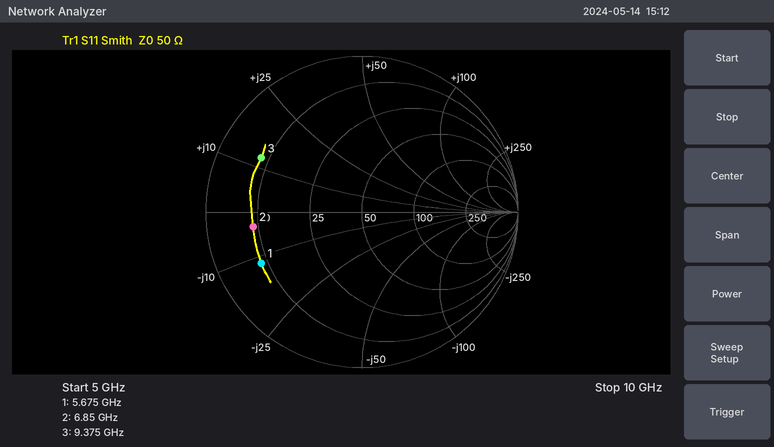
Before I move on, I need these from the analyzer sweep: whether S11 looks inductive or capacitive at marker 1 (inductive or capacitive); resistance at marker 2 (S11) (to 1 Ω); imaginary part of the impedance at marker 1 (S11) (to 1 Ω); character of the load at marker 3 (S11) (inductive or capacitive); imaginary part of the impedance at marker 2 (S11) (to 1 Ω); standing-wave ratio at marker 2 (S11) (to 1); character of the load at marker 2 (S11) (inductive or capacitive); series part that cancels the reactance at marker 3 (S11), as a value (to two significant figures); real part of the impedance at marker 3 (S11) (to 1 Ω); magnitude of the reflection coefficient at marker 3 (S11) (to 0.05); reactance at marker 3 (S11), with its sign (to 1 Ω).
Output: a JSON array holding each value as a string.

["capacitive", "9 Ω", "-12 Ω", "inductive", "-3 Ω", "6", "capacitive", "1.4 pF", "8 Ω", "0.75", "+12 Ω"]
